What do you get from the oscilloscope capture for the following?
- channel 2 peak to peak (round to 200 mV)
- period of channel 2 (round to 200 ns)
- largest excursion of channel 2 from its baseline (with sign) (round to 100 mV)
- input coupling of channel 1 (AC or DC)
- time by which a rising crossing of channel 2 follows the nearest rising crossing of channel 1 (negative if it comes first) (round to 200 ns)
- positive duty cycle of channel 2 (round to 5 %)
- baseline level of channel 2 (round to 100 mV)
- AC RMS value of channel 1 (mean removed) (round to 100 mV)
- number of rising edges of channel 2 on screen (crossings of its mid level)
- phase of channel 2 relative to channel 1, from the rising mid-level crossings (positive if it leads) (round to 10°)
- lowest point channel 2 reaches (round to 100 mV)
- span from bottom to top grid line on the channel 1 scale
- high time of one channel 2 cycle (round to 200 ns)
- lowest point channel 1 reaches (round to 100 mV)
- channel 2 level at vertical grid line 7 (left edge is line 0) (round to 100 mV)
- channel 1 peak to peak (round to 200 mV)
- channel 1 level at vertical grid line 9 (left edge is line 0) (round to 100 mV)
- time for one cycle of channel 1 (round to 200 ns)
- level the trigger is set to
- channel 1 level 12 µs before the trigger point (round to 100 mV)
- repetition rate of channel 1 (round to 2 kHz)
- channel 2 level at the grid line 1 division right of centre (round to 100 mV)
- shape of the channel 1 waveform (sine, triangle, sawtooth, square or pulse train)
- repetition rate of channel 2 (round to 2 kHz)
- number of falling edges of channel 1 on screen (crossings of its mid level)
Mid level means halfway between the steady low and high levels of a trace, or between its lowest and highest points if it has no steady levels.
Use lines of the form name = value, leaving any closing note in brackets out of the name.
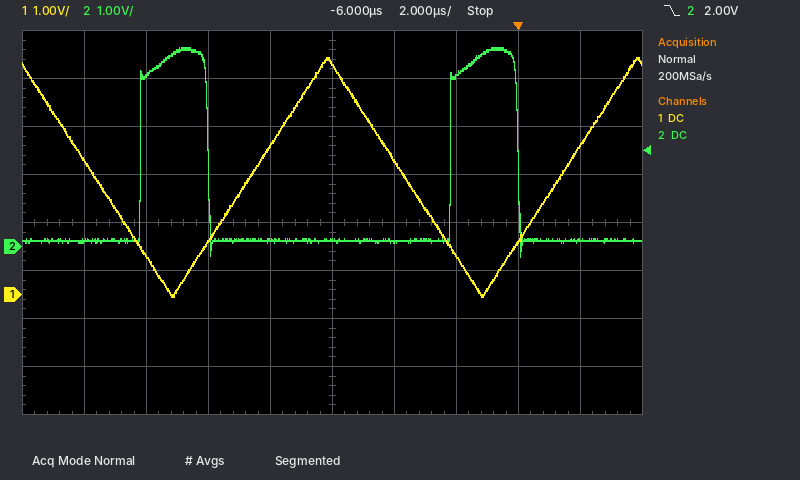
channel 2 peak to peak = 4.4 V
period of channel 2 = 10.0 µs
largest excursion of channel 2 from its baseline (with sign) = +4.0 V
input coupling of channel 1 = DC
time by which a rising crossing of channel 2 follows the nearest rising crossing of channel 1 (negative if it comes first) = -3.6 µs
positive duty cycle of channel 2 = 20 %
baseline level of channel 2 = 100 mV
AC RMS value of channel 1 (mean removed) = 1.4 V
number of rising edges of channel 2 on screen = 2
phase of channel 2 relative to channel 1, from the rising mid-level crossings (positive if it leads) = +130°
lowest point channel 2 reaches = -200 mV
span from bottom to top grid line on the channel 1 scale = 8 V
high time of one channel 2 cycle = 2.2 µs
lowest point channel 1 reaches = 0.0 V
channel 2 level at vertical grid line 7 (left edge is line 0) = 3.6 V
channel 1 peak to peak = 5.0 V
channel 1 level at vertical grid line 9 (left edge is line 0) = 3.1 V
time for one cycle of channel 1 = 10.0 µs
level the trigger is set to = 2.00 V
channel 1 level 12 µs before the trigger point = 800 mV
repetition rate of channel 1 = 100 kHz
channel 2 level at the grid line 1 division right of centre = 100 mV
shape of the channel 1 waveform = triangle
repetition rate of channel 2 = 100 kHz
number of falling edges of channel 1 on screen = 2
